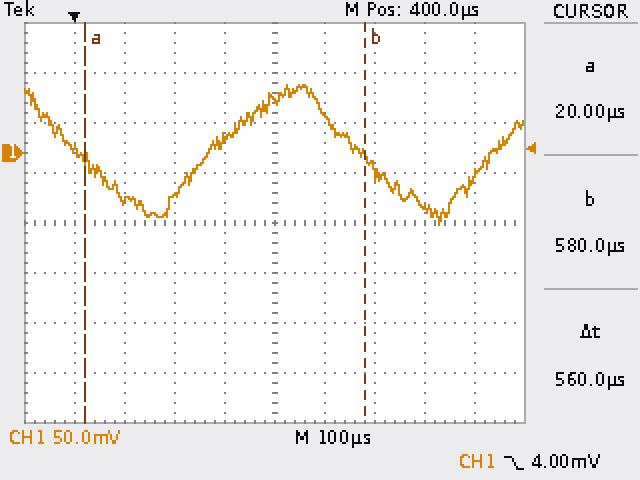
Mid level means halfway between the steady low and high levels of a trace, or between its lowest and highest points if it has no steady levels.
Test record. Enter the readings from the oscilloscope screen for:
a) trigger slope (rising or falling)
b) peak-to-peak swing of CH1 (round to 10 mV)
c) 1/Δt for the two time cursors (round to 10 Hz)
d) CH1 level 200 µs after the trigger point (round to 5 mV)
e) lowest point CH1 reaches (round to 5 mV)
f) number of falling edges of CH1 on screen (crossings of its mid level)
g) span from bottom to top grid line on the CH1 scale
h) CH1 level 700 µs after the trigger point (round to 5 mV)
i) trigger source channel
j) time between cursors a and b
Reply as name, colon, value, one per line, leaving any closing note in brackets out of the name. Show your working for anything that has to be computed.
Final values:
trigger slope: falling
peak-to-peak swing of CH1: 140 mV
1/Δt for the two time cursors: 1 / 560 µs ≈ 1.79 kHz
CH1 level 200 µs after the trigger point: -40 mV
lowest point CH1 reaches: -70 mV
number of falling edges of CH1 on screen: 2
span from bottom to top grid line on the CH1 scale: 400 mV
CH1 level 700 µs after the trigger point: -55 mV
trigger source channel: CH1
time between cursors a and b: 560 µs
